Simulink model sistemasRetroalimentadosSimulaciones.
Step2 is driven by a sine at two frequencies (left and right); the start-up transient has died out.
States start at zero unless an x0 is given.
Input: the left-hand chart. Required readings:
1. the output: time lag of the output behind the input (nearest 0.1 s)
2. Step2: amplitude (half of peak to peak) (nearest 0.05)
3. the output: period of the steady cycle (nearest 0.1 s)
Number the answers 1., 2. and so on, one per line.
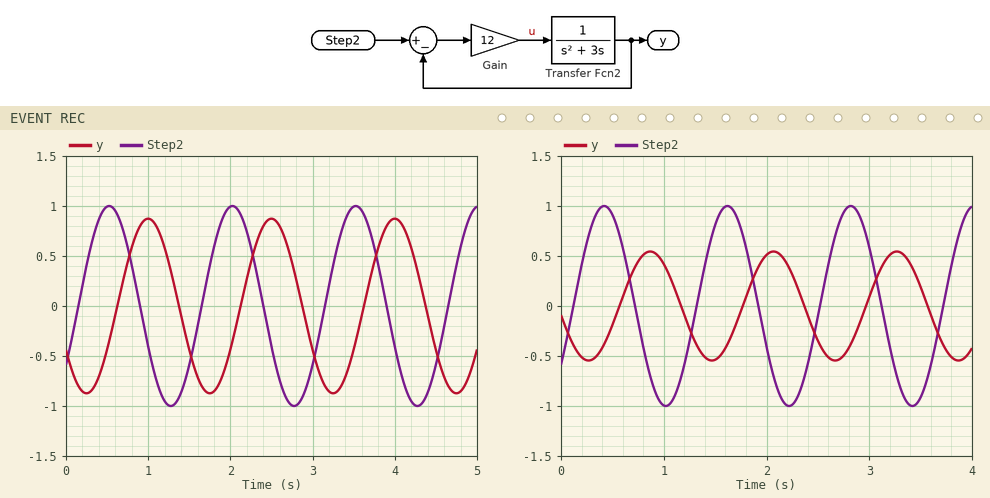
1. 0.5 s
2. 1.00
3. 1.5 s
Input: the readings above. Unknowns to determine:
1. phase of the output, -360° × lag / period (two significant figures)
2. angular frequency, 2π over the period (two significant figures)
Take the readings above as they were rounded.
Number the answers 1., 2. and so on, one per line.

1. -120°
2. 4.2 rad/s
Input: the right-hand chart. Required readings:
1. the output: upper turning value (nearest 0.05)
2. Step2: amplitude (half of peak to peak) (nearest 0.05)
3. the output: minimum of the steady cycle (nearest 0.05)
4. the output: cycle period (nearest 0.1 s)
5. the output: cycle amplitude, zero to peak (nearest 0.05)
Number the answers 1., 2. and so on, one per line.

1. 0.55
2. 1.00
3. -0.55
4. 1.2 s
5. 0.55
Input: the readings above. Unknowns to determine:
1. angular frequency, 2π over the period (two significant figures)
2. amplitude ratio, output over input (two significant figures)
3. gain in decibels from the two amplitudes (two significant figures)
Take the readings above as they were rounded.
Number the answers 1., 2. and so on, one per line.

1. 5.2 rad/s
2. 0.55
3. -5.2 dB
